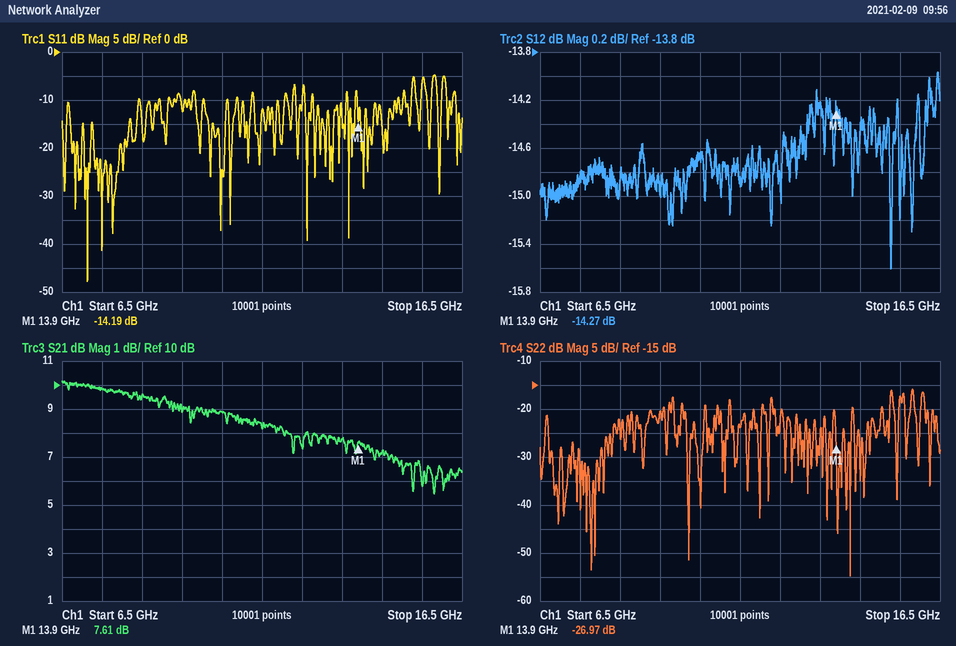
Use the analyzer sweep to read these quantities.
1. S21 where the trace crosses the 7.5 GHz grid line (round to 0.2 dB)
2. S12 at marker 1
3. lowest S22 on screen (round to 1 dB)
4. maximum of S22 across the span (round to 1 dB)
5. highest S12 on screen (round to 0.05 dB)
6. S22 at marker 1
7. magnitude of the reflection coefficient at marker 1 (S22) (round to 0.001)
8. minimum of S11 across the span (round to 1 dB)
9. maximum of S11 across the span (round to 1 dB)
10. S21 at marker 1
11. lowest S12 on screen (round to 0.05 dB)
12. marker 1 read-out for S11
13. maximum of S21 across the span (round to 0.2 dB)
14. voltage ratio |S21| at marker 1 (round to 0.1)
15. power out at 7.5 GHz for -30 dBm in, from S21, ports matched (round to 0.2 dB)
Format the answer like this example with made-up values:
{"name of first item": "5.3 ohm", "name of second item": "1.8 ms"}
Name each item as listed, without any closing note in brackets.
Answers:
{"S21 where the trace crosses the 7.5 GHz grid line": "9.8 dB", "S12 at marker 1": "-14.27 dB", "lowest S22 on screen": "-55 dB", "maximum of S22 across the span": "-16 dB", "highest S12 on screen": "-13.95 dB", "S22 at marker 1": "-26.97 dB", "magnitude of the reflection coefficient at marker 1 (S22)": "0.045", "minimum of S11 across the span": "-48 dB", "maximum of S11 across the span": "-5 dB", "S21 at marker 1": "7.61 dB", "lowest S12 on screen": "-15.60 dB", "marker 1 read-out for S11": "-14.19 dB", "maximum of S21 across the span": "10.2 dB", "voltage ratio |S21| at marker 1": "2.4", "power out at 7.5 GHz for -30 dBm in, from S21, ports matched": "-20.2 dBm"}
